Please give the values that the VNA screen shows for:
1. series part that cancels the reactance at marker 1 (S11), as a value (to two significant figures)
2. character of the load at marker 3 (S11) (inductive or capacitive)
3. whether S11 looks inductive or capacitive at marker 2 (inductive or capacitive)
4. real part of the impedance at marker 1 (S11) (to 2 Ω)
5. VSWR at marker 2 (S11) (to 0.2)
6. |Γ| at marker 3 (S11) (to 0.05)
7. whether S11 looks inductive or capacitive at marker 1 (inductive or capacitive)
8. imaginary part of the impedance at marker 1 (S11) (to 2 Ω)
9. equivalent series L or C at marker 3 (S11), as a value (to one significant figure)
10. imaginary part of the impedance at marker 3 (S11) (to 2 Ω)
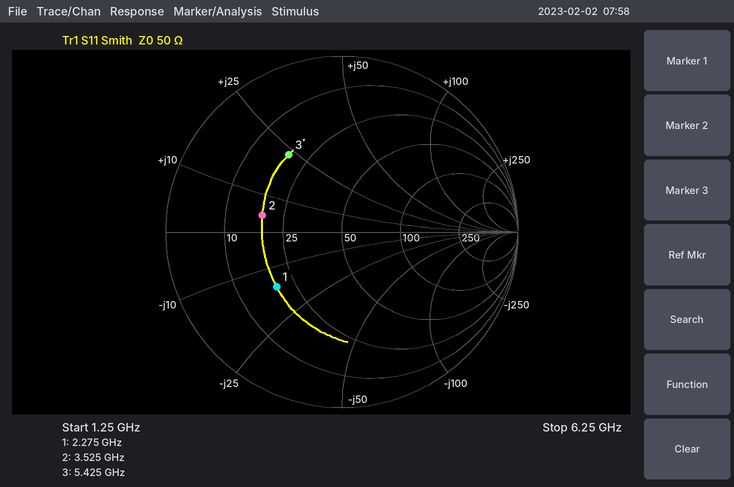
1.1 nH
inductive
inductive
20 Ω
2.8
0.55
capacitive
-16 Ω
700 pH
+24 Ω
